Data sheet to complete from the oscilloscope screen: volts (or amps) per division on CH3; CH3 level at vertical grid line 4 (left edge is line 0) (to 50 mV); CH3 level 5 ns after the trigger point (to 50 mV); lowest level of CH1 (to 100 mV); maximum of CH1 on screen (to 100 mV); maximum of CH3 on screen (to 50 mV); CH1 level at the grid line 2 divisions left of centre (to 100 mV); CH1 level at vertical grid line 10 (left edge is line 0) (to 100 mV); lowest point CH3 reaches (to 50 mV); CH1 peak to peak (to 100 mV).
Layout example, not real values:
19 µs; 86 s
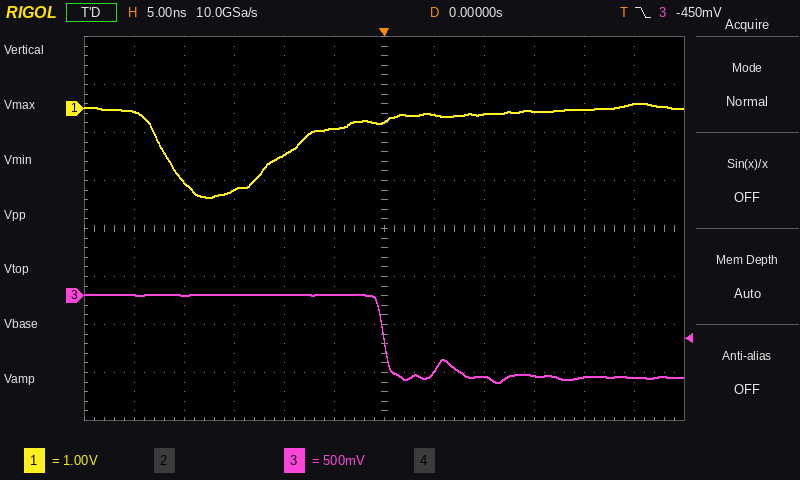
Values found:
500 mV; 0 mV; -800 mV; -1.9 V; 100 mV; 0 mV; -1.0 V; 0.0 V; -900 mV; 2.0 V
